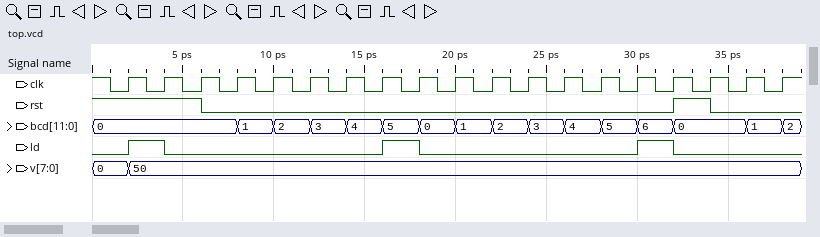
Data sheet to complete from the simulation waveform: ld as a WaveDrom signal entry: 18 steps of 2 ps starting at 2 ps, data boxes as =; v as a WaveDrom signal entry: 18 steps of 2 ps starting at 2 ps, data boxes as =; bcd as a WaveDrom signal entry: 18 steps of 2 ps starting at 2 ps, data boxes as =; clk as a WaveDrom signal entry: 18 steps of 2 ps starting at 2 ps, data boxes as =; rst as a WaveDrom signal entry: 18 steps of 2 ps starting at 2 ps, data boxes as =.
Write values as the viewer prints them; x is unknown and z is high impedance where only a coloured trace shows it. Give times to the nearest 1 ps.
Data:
{name: 'ld', wave: '10.....10.....10..'}
{name: 'v', wave: '=.................', data: '50'}
{name: 'bcd', wave: '=..=============.=', data: '0 1 2 3 4 5 0 1 2 3 4 5 6 0 1'}
{name: 'clk', wave: 'p.................'}
{name: 'rst', wave: '1.0............10.'}
